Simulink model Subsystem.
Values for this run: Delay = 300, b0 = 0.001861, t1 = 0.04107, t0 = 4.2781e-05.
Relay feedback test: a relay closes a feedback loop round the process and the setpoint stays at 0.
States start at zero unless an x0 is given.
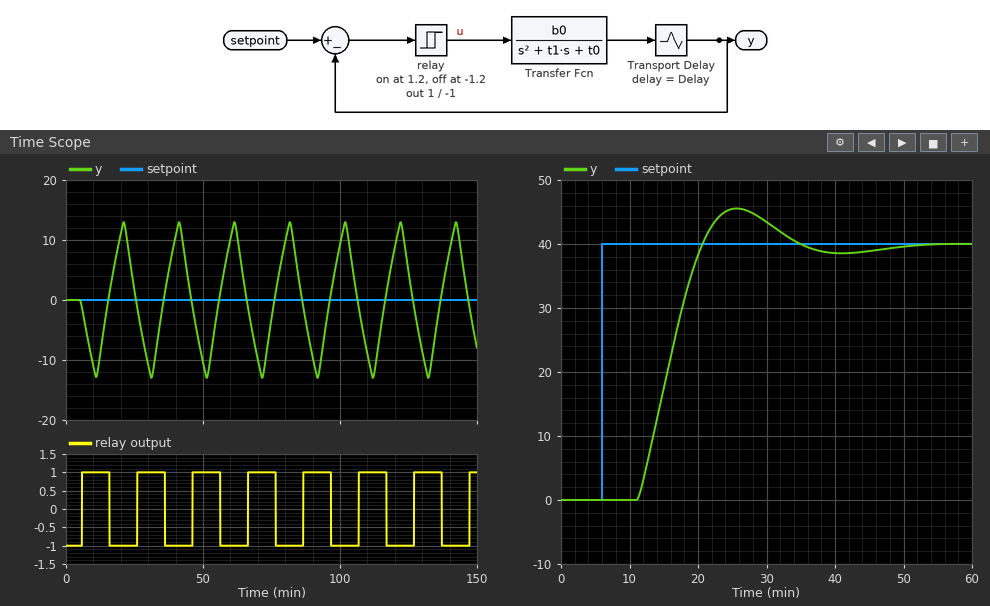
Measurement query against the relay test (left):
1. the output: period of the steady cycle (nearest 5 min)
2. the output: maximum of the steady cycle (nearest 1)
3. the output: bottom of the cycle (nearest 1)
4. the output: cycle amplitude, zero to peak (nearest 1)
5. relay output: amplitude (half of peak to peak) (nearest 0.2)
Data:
20 min
13
-13
13
1.0
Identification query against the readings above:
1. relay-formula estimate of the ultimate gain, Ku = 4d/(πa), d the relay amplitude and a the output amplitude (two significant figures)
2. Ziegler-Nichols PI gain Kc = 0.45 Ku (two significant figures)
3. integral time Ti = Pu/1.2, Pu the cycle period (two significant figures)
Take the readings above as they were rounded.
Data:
0.098
0.044
17 min
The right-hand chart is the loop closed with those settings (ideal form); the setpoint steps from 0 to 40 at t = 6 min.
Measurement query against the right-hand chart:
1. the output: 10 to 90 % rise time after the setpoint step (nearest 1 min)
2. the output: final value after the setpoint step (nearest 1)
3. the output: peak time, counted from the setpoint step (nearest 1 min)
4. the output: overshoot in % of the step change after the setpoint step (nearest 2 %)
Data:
7 min
40
20 min
14 %
